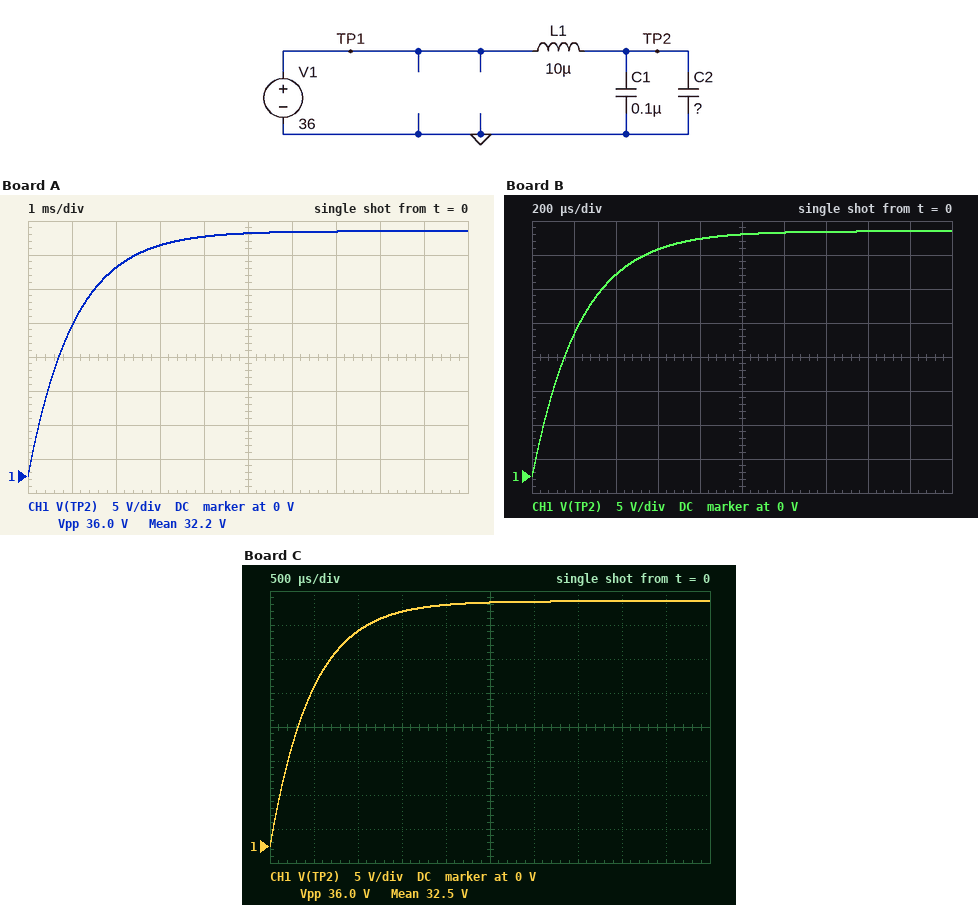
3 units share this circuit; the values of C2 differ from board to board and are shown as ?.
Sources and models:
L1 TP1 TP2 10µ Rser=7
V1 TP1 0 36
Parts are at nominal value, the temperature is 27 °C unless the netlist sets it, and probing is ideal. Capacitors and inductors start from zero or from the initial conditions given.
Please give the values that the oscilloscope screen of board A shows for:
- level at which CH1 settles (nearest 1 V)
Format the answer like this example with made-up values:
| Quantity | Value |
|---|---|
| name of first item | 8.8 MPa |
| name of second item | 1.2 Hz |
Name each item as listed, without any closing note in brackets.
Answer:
| Quantity | Value |
|---|---|
| level at which CH1 settles | 36 V |
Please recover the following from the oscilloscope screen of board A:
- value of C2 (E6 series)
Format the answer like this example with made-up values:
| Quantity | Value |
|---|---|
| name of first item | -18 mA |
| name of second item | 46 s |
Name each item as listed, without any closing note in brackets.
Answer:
| Quantity | Value |
|---|---|
| value of C2 | 150 µF |
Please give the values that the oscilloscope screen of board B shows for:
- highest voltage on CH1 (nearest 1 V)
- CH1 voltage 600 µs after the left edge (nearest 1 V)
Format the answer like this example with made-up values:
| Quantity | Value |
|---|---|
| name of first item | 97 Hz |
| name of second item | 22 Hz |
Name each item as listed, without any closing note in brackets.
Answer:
| Quantity | Value |
|---|---|
| highest voltage on CH1 | 36 V |
| CH1 voltage 600 µs after the left edge | 33 V |
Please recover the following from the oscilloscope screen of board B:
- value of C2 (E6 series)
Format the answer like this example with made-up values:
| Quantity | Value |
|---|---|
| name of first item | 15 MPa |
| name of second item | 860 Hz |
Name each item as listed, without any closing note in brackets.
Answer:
| Quantity | Value |
|---|---|
| value of C2 | 33 µF |
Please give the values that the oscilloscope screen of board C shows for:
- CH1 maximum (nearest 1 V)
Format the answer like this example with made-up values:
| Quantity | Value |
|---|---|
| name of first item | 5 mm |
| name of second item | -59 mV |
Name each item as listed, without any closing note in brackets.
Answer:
| Quantity | Value |
|---|---|
| CH1 maximum | 36 V |
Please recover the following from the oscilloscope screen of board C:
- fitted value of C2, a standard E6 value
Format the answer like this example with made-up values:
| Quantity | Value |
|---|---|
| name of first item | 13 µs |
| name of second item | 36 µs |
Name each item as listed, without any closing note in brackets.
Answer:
| Quantity | Value |
|---|---|
| fitted value of C2, a standard E6 value | 68 µF |
